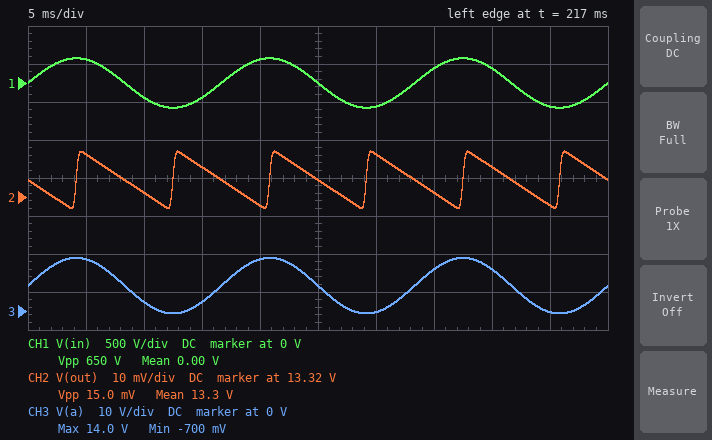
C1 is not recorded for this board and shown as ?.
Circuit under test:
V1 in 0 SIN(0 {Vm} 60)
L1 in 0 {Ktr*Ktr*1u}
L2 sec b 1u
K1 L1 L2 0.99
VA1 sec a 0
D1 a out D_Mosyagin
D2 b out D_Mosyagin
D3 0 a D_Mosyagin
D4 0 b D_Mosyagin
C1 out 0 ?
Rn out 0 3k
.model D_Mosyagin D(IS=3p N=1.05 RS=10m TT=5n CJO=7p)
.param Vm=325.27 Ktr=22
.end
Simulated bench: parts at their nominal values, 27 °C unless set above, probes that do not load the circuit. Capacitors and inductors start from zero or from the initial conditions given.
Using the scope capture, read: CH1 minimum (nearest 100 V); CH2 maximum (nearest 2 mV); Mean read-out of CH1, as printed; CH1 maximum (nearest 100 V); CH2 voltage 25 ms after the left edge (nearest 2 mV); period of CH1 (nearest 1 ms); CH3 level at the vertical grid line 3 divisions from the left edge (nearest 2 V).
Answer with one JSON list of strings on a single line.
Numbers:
["-300 V", "13.332 V", "0.00 V", "300 V", "13.324 V", "17 ms", "2 V"]
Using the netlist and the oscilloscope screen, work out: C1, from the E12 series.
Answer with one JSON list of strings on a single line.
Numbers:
["2.2 mF"]
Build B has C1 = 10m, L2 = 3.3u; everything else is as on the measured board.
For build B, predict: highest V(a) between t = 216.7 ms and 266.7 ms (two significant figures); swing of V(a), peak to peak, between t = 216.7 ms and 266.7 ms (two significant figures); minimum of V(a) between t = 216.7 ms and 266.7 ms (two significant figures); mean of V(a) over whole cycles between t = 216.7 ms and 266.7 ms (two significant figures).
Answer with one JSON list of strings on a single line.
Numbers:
["26 V", "27 V", "-680 mV", "13 V"]
